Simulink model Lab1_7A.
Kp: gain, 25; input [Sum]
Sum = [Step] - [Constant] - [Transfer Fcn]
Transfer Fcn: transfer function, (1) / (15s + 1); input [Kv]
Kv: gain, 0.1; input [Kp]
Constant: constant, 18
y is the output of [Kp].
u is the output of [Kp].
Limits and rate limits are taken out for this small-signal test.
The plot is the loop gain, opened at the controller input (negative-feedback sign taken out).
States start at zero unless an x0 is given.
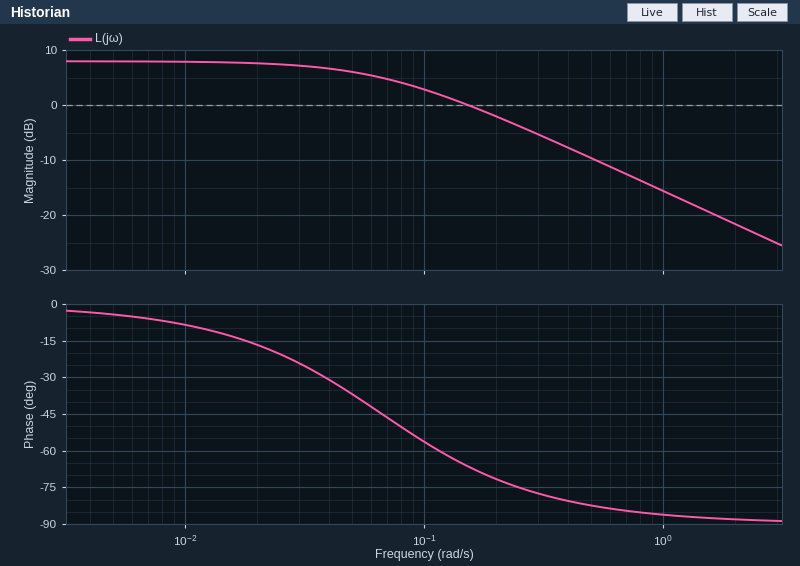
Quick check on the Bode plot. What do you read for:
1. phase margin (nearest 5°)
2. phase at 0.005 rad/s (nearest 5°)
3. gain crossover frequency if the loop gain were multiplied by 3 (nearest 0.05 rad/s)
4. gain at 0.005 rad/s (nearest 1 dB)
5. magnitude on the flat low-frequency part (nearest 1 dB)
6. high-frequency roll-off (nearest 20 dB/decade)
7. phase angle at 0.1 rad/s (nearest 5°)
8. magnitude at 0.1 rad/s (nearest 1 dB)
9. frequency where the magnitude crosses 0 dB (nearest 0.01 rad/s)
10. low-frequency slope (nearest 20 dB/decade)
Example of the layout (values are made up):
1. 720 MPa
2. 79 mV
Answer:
1. 115°
2. -5°
3. 0.50 rad/s
4. 8 dB
5. 8 dB
6. -20 dB/decade
7. -55°
8. 3 dB
9. 0.15 rad/s
10. 0 dB/decade
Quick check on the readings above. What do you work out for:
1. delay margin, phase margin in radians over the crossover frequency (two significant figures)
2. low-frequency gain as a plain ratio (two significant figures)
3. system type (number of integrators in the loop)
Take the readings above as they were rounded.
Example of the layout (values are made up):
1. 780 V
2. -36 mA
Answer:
1. 13 s
2. 2.5
3. 0
